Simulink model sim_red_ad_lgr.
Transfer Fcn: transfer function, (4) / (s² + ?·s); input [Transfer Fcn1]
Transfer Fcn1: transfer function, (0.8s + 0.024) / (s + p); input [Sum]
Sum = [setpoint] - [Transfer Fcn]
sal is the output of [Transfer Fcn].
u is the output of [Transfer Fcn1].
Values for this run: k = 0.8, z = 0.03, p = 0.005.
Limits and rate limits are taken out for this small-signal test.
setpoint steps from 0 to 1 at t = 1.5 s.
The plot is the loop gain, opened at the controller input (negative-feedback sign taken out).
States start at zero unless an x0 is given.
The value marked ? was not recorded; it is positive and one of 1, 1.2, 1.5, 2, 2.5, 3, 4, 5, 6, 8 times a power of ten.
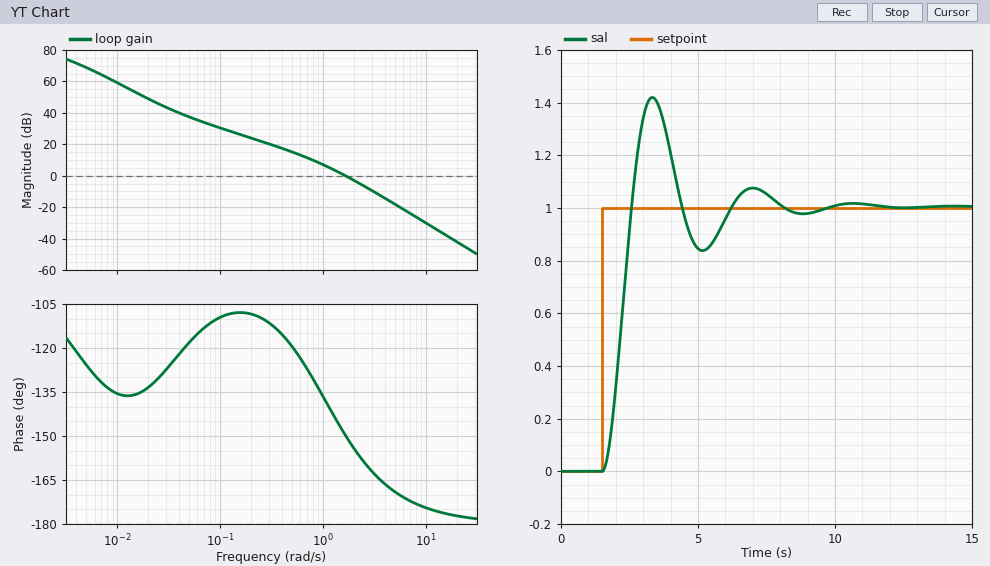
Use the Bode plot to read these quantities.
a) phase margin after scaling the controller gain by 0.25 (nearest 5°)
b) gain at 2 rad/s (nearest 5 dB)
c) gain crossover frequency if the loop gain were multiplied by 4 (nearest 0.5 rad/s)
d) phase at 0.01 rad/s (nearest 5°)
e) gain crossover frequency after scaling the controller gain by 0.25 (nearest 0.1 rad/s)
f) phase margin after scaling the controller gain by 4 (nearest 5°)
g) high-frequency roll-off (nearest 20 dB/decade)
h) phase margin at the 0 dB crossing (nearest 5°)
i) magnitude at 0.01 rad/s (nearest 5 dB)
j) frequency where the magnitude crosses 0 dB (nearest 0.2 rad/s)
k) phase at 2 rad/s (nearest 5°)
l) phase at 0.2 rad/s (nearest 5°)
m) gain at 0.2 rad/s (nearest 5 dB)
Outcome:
55°
-5 dB
3.5 rad/s
-135°
0.7 rad/s
15°
-40 dB/decade
30°
60 dB
1.6 rad/s
-155°
-110°
25 dB
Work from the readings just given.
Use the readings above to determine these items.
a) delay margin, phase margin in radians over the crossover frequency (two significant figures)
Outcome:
0.33 s
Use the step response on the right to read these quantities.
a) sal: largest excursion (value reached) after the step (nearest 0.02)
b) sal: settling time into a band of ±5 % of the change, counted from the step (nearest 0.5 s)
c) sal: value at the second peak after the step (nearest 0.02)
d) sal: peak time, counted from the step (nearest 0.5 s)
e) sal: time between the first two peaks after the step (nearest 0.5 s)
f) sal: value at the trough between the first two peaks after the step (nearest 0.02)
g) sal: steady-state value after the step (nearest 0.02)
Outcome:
1.42
6.0 s
1.08
2.0 s
3.5 s
0.84
1.00
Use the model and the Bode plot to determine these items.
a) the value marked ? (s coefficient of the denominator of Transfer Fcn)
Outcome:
1
